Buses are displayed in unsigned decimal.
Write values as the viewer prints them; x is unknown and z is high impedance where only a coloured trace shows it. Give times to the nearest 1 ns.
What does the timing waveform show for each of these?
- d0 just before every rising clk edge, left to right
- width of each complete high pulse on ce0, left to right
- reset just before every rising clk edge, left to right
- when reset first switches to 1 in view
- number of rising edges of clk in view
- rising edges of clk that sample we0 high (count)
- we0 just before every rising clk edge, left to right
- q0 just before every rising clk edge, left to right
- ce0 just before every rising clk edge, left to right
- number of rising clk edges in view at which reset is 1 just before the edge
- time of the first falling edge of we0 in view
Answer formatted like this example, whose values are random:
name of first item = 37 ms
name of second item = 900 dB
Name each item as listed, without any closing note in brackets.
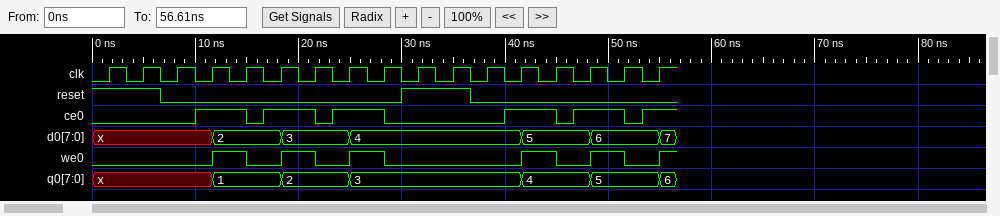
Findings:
d0 just before every rising clk edge, left to right = x, x, x, x, 2, 2, 3, 3, 4, 4, 4, 4, 4, 5, 5, 6, 6
width of each complete high pulse on ce0, left to right = 5 ns, 5 ns, 5 ns, 5 ns, 5 ns
reset just before every rising clk edge, left to right = 1 1 0 0 0 0 0 0 0 1 1 0 0 0 0 0 0
when reset first switches to 1 in view = 30 ns
number of rising edges of clk in view = 17
rising edges of clk that sample we0 high = 5
we0 just before every rising clk edge, left to right = 0 0 0 0 1 0 1 0 1 0 0 0 0 1 0 1 0
q0 just before every rising clk edge, left to right = x, x, x, x, 1, 1, 2, 2, 3, 3, 3, 3, 3, 4, 4, 5, 5
ce0 just before every rising clk edge, left to right = 0 0 0 1 1 1 1 1 1 0 0 0 1 1 1 1 1
number of rising clk edges in view at which reset is 1 just before the edge = 4
time of the first falling edge of we0 in view = 15 ns
